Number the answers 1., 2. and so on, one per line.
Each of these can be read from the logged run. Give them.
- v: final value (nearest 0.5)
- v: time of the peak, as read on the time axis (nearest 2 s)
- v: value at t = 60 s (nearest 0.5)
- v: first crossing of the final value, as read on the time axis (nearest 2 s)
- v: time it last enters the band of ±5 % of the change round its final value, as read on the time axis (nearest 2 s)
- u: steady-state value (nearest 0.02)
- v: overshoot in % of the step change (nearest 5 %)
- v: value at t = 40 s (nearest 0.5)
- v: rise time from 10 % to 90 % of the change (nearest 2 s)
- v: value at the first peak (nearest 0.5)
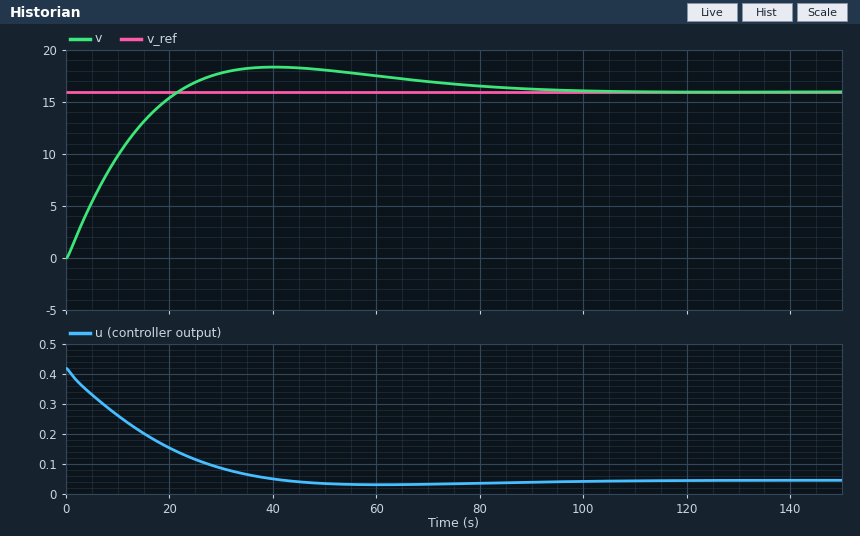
1. 16.0
2. 40 s
3. 17.5
4. 22 s
5. 74 s
6. 0.04
7. 15 %
8. 18.5
9. 16 s
10. 18.5
